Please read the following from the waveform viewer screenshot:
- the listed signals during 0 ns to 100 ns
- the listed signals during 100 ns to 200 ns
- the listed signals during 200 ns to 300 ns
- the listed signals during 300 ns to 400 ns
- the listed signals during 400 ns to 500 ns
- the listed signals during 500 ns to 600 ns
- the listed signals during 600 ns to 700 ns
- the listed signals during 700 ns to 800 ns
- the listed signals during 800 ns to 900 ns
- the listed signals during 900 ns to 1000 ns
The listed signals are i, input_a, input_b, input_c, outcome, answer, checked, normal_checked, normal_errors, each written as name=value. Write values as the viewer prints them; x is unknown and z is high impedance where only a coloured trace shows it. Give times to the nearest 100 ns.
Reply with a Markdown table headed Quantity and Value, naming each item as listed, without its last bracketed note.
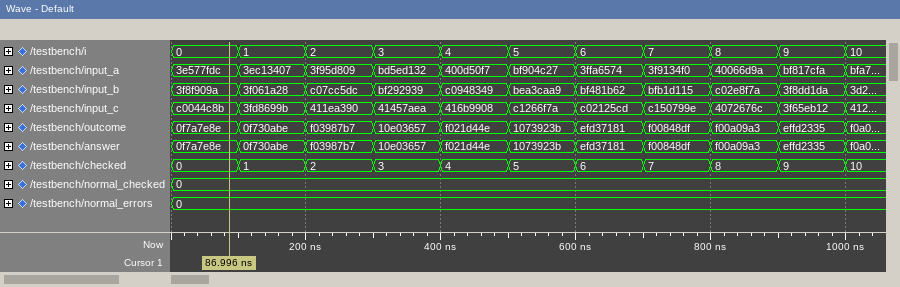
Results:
| Quantity | Value |
|---|---|
| the listed signals during 0 ns to 100 ns | i=0, input_a=3e577fdc, input_b=3f8f909a, input_c=c0044c8b, outcome=0f7a7e8e, answer=0f7a7e8e, checked=0, normal_checked=0, normal_errors=0 |
| the listed signals during 100 ns to 200 ns | i=1, input_a=3ec13407, input_b=3f061a28, input_c=3fd8699b, outcome=0f730abe, answer=0f730abe, checked=1, normal_checked=0, normal_errors=0 |
| the listed signals during 200 ns to 300 ns | i=2, input_a=3f95d809, input_b=c07cc5dc, input_c=411ea390, outcome=f03987b7, answer=f03987b7, checked=2, normal_checked=0, normal_errors=0 |
| the listed signals during 300 ns to 400 ns | i=3, input_a=bd5ed132, input_b=bf292939, input_c=41457aea, outcome=10e03657, answer=10e03657, checked=3, normal_checked=0, normal_errors=0 |
| the listed signals during 400 ns to 500 ns | i=4, input_a=400d50f7, input_b=c0948349, input_c=416b9908, outcome=f021d44e, answer=f021d44e, checked=4, normal_checked=0, normal_errors=0 |
| the listed signals during 500 ns to 600 ns | i=5, input_a=bf904c27, input_b=bea3caa9, input_c=c1266f7a, outcome=1073923b, answer=1073923b, checked=5, normal_checked=0, normal_errors=0 |
| the listed signals during 600 ns to 700 ns | i=6, input_a=3ffa6574, input_b=bf481b62, input_c=c02125cd, outcome=efd37181, answer=efd37181, checked=6, normal_checked=0, normal_errors=0 |
| the listed signals during 700 ns to 800 ns | i=7, input_a=3f9134f0, input_b=bfb1d115, input_c=c150799e, outcome=f00848df, answer=f00848df, checked=7, normal_checked=0, normal_errors=0 |
| the listed signals during 800 ns to 900 ns | i=8, input_a=40066d9a, input_b=c02e8f7a, input_c=4072676c, outcome=f00a09a3, answer=f00a09a3, checked=8, normal_checked=0, normal_errors=0 |
| the listed signals during 900 ns to 1000 ns | i=9, input_a=bf817cfa, input_b=3f8dd1da, input_c=3f65eb12, outcome=effd2335, answer=effd2335, checked=9, normal_checked=0, normal_errors=0 |
